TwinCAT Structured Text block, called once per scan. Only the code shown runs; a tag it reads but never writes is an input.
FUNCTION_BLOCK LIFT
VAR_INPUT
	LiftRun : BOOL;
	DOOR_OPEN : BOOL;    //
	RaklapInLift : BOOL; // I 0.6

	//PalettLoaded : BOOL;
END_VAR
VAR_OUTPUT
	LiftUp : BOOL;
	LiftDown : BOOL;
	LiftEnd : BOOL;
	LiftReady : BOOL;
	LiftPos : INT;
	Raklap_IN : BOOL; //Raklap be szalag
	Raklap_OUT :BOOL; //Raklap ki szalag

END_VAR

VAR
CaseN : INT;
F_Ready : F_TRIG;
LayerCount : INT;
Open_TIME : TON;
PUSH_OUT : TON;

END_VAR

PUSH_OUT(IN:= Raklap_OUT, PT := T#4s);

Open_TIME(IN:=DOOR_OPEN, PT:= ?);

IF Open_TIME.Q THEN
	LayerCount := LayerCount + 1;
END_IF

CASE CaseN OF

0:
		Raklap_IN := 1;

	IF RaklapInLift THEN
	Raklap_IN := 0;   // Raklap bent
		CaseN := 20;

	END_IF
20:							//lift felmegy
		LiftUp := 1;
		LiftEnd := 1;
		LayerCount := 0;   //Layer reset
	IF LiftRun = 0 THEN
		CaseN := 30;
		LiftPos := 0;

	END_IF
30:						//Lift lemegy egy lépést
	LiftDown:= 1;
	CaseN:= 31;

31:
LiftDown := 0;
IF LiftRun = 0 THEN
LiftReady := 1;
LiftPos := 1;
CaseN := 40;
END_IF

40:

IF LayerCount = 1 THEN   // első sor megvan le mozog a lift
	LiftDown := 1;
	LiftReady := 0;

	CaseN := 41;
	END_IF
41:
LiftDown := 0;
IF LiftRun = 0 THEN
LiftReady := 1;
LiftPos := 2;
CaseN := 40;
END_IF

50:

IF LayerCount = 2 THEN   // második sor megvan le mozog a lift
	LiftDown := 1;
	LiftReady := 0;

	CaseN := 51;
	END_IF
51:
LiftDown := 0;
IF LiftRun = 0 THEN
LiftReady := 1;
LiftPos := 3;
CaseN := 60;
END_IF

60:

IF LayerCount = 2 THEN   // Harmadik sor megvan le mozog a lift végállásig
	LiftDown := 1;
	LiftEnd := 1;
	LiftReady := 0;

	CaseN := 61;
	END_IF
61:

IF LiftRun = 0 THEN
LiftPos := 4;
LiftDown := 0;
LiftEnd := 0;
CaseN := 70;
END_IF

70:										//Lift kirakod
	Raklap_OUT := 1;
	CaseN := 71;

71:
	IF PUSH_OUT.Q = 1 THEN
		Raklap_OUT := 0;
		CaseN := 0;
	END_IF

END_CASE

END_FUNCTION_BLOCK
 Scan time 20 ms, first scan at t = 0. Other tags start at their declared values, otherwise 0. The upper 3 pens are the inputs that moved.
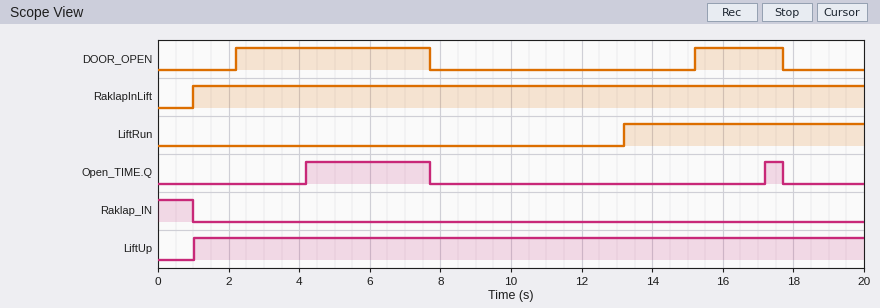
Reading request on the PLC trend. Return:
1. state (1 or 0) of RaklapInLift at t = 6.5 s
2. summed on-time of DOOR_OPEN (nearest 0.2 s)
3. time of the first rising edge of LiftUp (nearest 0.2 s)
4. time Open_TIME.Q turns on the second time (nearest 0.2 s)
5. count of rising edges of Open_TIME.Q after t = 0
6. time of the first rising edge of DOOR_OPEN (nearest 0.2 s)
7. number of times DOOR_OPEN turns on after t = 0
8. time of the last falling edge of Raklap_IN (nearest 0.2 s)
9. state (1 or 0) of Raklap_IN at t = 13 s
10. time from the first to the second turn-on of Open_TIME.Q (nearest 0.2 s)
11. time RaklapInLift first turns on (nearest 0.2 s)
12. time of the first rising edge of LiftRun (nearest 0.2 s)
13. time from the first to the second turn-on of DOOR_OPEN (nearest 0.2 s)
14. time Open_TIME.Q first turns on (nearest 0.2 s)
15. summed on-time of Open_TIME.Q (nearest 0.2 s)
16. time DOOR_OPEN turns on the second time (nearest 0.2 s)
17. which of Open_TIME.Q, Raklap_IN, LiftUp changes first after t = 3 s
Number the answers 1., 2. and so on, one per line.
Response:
1. 1
2. 8.0 s
3. 1.0 s
4. 17.2 s
5. 2
6. 2.2 s
7. 2
8. 1.0 s
9. 0
10. 13.0 s
11. 1.0 s
12. 13.2 s
13. 13.0 s
14. 4.2 s
15. 4.0 s
16. 15.2 s
17. Open_TIME.Q
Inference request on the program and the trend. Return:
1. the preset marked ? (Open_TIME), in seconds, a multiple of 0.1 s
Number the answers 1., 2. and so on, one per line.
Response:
1. 2.0 s
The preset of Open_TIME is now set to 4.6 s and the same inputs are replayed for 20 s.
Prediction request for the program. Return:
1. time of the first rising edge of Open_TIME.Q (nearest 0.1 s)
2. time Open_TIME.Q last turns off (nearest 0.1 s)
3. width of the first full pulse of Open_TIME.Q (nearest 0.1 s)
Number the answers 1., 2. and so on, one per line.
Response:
1. 6.8 s
2. 7.7 s
3. 0.9 s
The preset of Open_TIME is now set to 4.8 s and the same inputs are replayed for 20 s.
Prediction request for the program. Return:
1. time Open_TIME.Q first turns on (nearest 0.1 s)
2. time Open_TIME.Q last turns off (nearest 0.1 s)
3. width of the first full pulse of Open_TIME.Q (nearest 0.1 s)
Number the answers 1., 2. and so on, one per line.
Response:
1. 7.0 s
2. 7.7 s
3. 0.7 s
